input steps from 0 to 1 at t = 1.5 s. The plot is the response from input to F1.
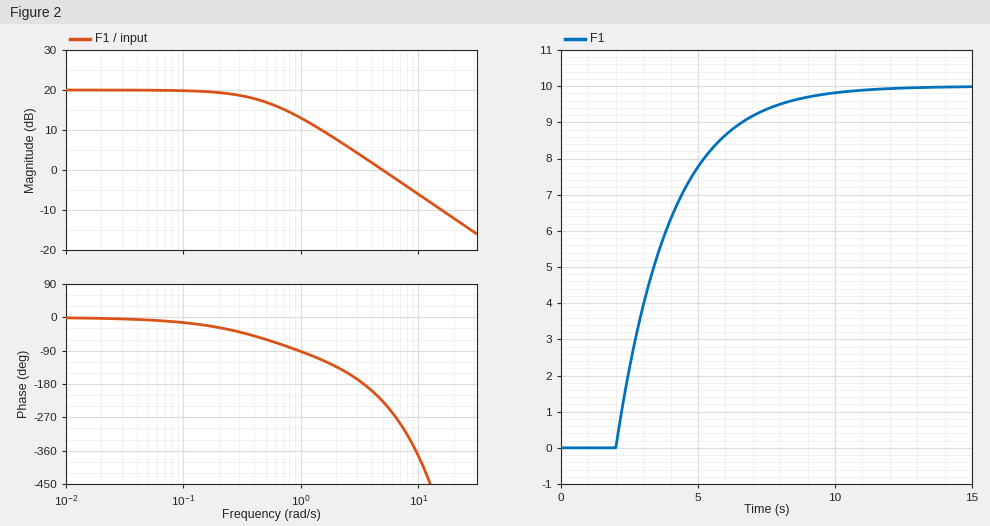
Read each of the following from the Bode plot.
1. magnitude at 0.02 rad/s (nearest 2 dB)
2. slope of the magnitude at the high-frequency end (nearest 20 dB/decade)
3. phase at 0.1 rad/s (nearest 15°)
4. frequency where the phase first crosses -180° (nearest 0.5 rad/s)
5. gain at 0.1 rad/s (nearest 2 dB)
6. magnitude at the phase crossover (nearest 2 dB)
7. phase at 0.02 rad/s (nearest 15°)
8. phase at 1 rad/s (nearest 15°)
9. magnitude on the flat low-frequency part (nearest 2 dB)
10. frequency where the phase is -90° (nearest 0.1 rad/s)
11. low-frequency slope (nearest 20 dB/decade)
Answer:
20 dB
-20 dB/decade
-15°
3.5 rad/s
20 dB
4 dB
0°
-90°
20 dB
1.0 rad/s
0 dB/decade
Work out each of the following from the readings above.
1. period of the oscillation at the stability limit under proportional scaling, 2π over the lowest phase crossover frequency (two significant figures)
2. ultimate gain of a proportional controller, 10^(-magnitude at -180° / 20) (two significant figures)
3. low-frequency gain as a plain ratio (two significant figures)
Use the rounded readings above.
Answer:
1.8 s
0.63
10
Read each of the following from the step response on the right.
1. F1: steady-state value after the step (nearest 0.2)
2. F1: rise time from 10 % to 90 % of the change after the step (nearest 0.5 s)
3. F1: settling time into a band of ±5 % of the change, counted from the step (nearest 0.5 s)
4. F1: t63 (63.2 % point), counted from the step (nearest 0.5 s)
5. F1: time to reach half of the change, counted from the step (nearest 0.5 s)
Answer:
10.0
4.5 s
6.5 s
2.5 s
2.0 s
